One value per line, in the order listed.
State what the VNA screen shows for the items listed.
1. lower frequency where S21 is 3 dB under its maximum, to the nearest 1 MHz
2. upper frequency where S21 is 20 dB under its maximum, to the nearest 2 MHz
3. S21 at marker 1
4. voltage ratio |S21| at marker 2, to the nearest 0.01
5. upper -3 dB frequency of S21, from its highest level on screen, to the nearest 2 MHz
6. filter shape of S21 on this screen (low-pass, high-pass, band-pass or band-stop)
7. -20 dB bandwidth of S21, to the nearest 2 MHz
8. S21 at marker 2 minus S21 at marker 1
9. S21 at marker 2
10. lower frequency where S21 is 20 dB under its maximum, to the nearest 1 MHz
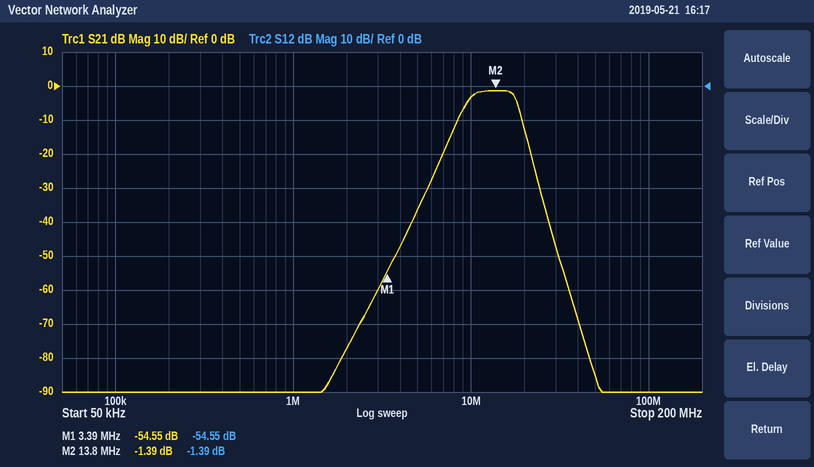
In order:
10 MHz
22 MHz
-54.55 dB
0.85
18 MHz
band-pass
16 MHz
53.16 dB
-1.39 dB
7 MHz
